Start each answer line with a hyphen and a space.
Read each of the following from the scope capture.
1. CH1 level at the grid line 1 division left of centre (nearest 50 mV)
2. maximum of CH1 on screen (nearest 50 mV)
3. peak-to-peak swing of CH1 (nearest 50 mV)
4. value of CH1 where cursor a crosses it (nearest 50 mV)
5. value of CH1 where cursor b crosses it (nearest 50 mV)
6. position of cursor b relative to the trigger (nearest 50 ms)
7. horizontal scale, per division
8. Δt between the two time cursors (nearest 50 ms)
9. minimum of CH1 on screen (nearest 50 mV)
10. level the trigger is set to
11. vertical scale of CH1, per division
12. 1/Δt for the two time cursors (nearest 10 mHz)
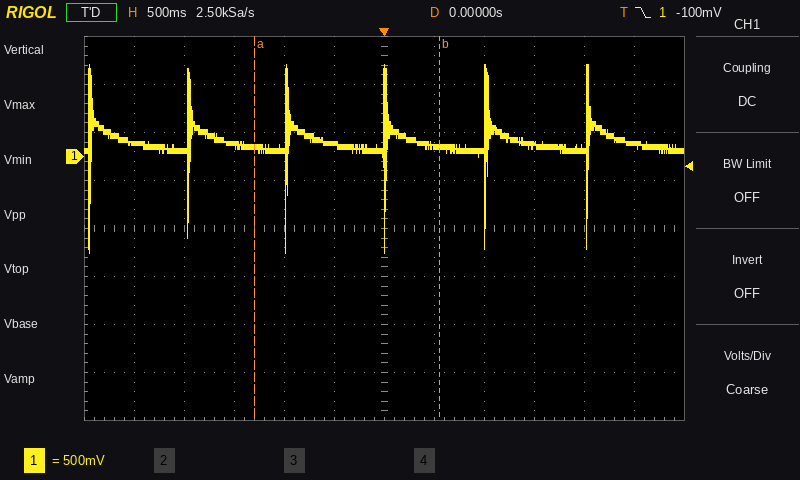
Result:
- 150 mV
- 950 mV
- 1.95 V
- 100 mV
- 100 mV
- +550 ms
- 500 ms
- 1.85 s
- -1.00 V
- -100 mV
- 500 mV
- 540 mHz
